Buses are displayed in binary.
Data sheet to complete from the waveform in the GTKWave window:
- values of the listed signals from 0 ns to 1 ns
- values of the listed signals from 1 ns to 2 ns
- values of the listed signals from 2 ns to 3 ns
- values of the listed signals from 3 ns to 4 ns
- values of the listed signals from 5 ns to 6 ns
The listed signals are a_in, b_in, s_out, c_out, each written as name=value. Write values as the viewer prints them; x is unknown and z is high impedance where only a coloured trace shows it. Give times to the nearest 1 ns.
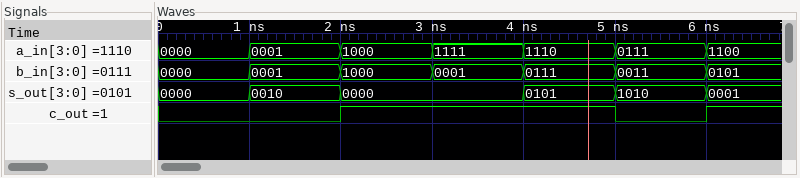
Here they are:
a_in=0000, b_in=0000, s_out=0000, c_out=0
a_in=0001, b_in=0001, s_out=0010, c_out=0
a_in=1000, b_in=1000, s_out=0000, c_out=1
a_in=1111, b_in=0001, s_out=0000, c_out=1
a_in=0111, b_in=0011, s_out=1010, c_out=0
